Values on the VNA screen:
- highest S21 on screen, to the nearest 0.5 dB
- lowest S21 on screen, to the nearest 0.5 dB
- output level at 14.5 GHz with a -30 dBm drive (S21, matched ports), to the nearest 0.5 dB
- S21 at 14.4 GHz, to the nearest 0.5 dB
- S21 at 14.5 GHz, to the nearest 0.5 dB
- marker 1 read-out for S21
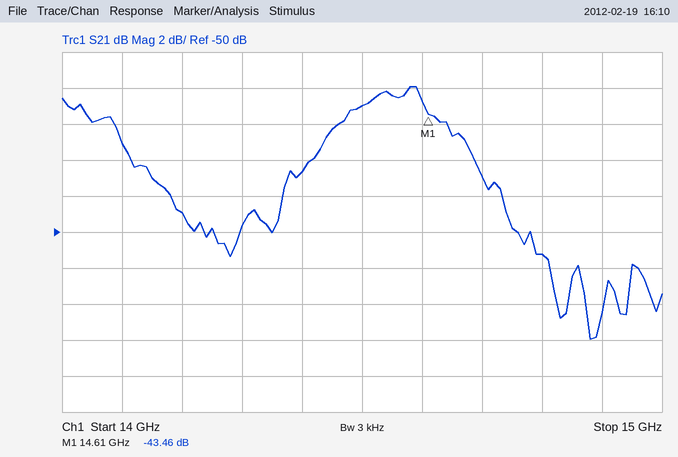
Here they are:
-42.0 dB
-56.0 dB
-73.0 dBm
-46.5 dB
-43.0 dB
-43.46 dB
